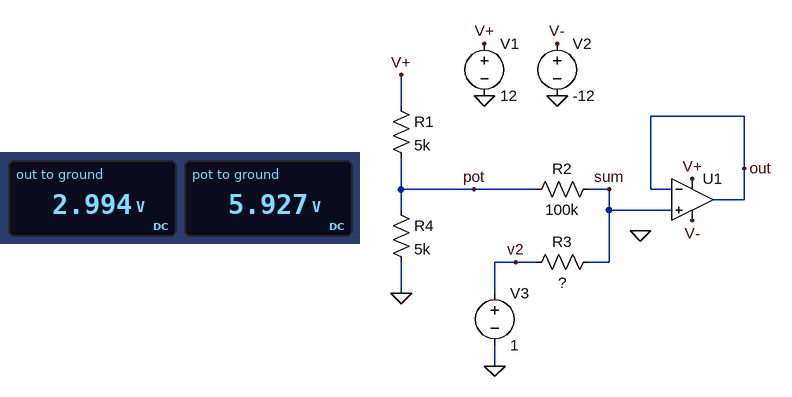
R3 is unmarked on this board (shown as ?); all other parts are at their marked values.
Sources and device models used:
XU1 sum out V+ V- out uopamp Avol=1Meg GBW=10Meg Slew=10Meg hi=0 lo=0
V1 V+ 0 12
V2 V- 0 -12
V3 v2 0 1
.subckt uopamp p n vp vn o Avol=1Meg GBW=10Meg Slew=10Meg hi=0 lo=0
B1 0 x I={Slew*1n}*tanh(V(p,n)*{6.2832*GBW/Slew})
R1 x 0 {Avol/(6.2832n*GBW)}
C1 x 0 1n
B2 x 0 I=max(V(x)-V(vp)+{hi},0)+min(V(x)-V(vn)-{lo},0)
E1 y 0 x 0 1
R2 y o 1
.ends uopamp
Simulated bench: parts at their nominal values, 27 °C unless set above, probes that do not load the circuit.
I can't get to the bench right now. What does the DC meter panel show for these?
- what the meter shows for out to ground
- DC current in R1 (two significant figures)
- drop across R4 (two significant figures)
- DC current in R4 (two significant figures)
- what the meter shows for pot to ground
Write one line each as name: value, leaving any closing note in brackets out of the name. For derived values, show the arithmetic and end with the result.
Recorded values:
what the meter shows for out to ground: 2.994 V
DC current in R1: (12 V - 5.927 V) / 5 kΩ = 1.2 mA
drop across R4: 5.927 V = 5.9 V
DC current in R4: (5.927 V) / 5 kΩ = 1.2 mA
what the meter shows for pot to ground: 5.927 V
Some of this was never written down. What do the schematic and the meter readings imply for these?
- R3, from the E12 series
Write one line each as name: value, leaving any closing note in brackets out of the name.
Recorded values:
R3, from the E12 series: 68 kΩ
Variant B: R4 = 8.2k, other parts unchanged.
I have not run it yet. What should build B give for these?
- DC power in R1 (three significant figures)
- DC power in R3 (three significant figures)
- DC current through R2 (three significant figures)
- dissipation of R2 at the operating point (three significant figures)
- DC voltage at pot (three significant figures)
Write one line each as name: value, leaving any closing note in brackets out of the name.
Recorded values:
DC power in R1: 4.35 mW
DC power in R3: 96.8 µW
DC current through R2: 37.7 µA
dissipation of R2 at the operating point: 142 µW
DC voltage at pot: 7.34 V
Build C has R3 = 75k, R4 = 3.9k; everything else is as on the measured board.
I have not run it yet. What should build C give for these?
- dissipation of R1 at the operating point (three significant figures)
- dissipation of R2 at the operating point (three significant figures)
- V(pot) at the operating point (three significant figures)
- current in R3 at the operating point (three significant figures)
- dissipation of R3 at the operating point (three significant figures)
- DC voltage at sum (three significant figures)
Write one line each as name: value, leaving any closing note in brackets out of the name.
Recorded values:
dissipation of R1 at the operating point: 9.23 mW
dissipation of R2 at the operating point: 57.8 µW
V(pot) at the operating point: 5.21 V
current in R3 at the operating point: 24.0 µA
dissipation of R3 at the operating point: 43.3 µW
DC voltage at sum: 2.80 V
